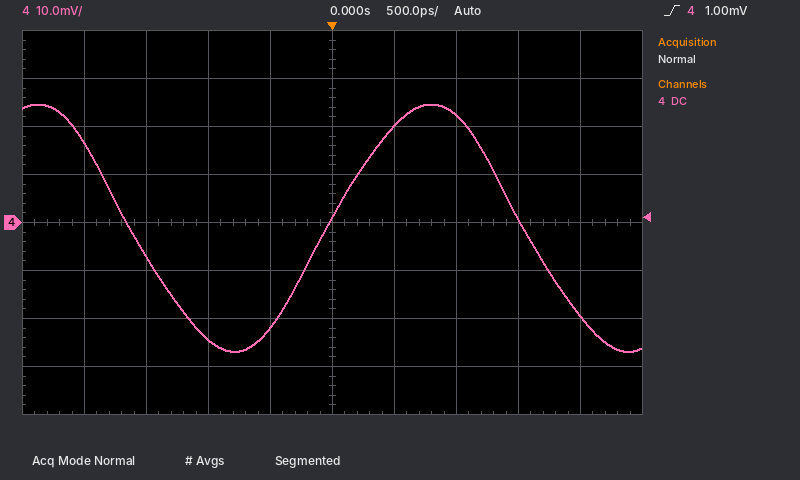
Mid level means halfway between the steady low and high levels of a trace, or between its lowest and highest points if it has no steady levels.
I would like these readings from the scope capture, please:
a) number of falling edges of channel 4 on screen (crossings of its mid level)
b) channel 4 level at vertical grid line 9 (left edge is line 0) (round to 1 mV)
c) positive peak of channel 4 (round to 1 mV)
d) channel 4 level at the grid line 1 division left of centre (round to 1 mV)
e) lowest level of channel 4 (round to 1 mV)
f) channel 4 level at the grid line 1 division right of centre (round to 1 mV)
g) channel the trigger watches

2
-19 mV
25 mV
-22 mV
-27 mV
20 mV
channel 4
